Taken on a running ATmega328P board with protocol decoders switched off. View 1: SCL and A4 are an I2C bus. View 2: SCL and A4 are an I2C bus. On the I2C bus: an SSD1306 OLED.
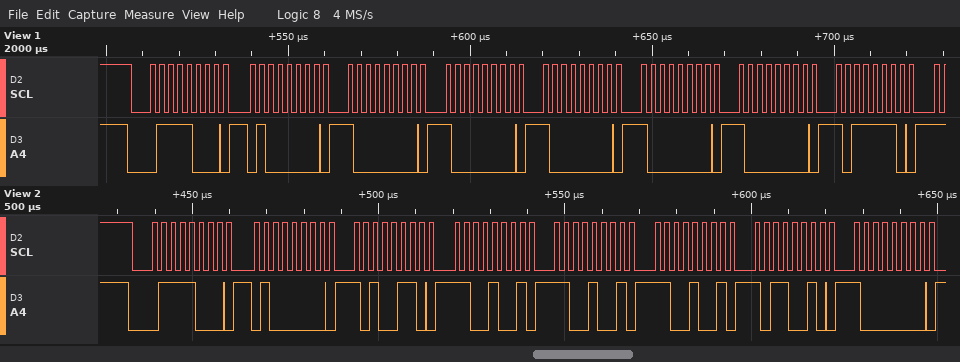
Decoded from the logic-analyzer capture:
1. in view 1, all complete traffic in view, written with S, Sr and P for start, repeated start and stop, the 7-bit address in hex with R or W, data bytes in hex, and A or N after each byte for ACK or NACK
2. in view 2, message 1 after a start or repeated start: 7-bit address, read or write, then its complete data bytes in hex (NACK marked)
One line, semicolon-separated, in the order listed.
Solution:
S 3CW A 40 A 80 A 80 A 80 A 80 A 80 A BE A; 0x3C write: 40 A6 C9 C9 C9 B2 80
